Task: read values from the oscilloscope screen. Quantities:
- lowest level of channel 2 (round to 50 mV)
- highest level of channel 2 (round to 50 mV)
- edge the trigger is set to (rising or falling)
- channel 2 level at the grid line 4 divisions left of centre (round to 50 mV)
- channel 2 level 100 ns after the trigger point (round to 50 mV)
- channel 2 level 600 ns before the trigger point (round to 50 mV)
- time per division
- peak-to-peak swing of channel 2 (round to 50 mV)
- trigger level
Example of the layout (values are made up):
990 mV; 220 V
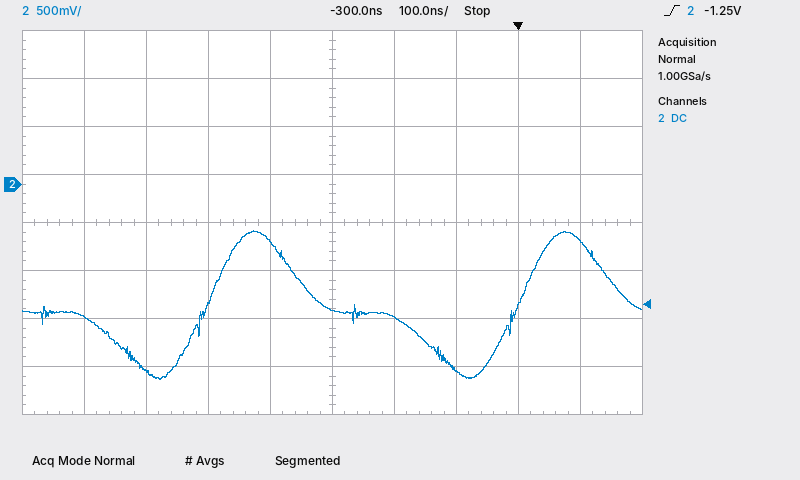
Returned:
-2.05 V; -500 mV; rising; -1.40 V; -600 mV; -1.95 V; 100 ns; 1.55 V; -1.25 V
